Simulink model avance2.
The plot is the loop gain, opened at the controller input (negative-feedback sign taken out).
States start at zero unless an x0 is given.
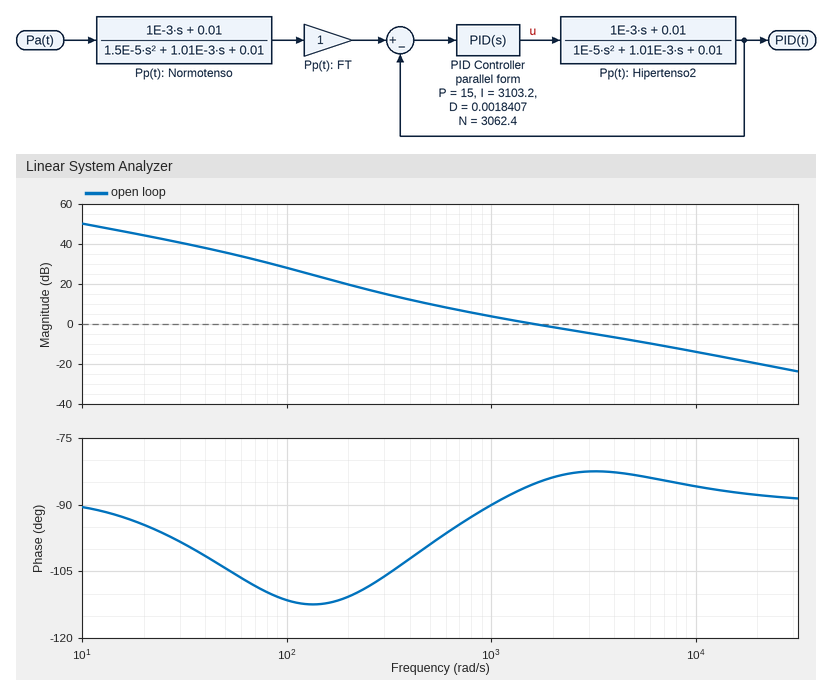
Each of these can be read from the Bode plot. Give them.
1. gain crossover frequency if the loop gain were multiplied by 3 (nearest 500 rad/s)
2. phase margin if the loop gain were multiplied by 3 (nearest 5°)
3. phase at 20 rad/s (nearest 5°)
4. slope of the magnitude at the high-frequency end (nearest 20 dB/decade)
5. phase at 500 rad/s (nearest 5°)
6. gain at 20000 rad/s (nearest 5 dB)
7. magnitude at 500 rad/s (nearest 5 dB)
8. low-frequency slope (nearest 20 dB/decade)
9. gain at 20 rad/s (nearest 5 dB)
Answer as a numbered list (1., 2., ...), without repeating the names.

1. 6000 rad/s
2. 95°
3. -95°
4. -20 dB/decade
5. -100°
6. -20 dB
7. 10 dB
8. -20 dB/decade
9. 45 dB
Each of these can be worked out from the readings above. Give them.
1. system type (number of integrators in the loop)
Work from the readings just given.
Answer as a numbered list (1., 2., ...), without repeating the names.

1. 1
